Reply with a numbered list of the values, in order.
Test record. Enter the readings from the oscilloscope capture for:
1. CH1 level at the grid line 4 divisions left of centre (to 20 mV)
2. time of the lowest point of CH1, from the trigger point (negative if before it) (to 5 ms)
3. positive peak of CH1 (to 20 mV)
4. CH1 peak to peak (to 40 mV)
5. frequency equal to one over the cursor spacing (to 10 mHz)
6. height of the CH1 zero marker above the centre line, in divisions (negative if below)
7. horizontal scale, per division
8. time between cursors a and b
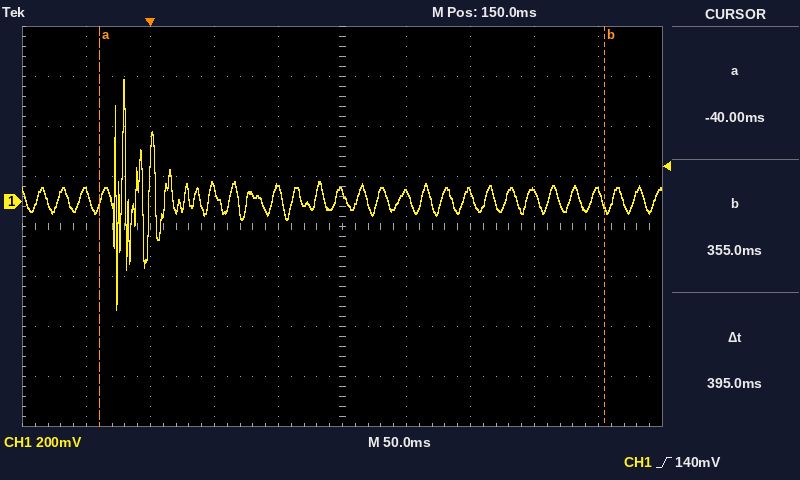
1. 40 mV
2. -25 ms
3. 480 mV
4. 920 mV
5. 2.53 Hz
6. +0.5 div
7. 50 ms
8. 395 ms
